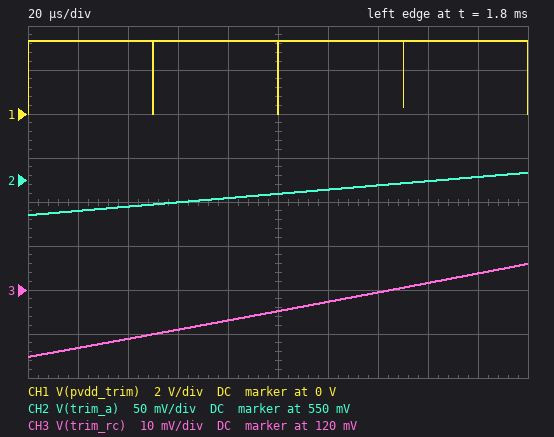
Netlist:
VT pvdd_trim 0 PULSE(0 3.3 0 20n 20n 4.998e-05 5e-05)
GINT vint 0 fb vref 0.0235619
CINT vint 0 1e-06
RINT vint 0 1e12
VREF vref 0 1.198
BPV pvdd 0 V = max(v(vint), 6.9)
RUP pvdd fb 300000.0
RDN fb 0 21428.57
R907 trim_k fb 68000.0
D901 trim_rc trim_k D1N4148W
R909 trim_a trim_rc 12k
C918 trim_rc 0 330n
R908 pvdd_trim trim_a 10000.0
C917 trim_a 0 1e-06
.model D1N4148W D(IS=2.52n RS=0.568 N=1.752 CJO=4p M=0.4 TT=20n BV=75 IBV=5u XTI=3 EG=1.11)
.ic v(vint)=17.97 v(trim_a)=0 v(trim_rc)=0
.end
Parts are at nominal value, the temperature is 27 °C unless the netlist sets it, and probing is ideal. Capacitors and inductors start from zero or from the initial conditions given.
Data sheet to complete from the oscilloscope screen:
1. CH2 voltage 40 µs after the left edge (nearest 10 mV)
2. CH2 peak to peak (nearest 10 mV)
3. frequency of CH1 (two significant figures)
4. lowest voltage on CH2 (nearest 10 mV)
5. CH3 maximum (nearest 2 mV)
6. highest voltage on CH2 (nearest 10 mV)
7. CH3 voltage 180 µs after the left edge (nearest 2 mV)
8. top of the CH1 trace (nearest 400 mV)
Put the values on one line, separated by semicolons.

520 mV; 50 mV; 20 kHz; 510 mV; 126 mV; 560 mV; 124 mV; 3.2 V
